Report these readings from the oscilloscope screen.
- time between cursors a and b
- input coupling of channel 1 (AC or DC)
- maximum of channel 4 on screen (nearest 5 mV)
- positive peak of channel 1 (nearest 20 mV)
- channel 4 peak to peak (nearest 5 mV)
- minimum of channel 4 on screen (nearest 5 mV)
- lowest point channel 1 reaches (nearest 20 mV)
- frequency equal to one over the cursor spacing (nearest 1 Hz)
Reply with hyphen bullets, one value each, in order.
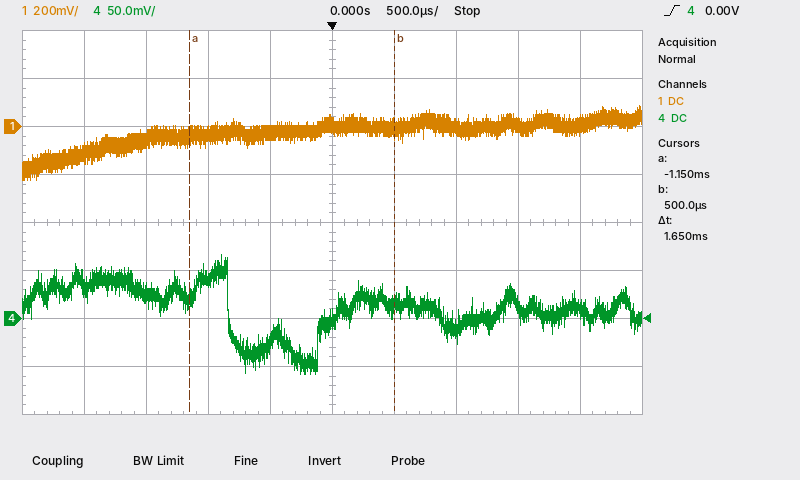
- 1.65 ms
- DC
- 65 mV
- 80 mV
- 125 mV
- -60 mV
- -220 mV
- 606 Hz
